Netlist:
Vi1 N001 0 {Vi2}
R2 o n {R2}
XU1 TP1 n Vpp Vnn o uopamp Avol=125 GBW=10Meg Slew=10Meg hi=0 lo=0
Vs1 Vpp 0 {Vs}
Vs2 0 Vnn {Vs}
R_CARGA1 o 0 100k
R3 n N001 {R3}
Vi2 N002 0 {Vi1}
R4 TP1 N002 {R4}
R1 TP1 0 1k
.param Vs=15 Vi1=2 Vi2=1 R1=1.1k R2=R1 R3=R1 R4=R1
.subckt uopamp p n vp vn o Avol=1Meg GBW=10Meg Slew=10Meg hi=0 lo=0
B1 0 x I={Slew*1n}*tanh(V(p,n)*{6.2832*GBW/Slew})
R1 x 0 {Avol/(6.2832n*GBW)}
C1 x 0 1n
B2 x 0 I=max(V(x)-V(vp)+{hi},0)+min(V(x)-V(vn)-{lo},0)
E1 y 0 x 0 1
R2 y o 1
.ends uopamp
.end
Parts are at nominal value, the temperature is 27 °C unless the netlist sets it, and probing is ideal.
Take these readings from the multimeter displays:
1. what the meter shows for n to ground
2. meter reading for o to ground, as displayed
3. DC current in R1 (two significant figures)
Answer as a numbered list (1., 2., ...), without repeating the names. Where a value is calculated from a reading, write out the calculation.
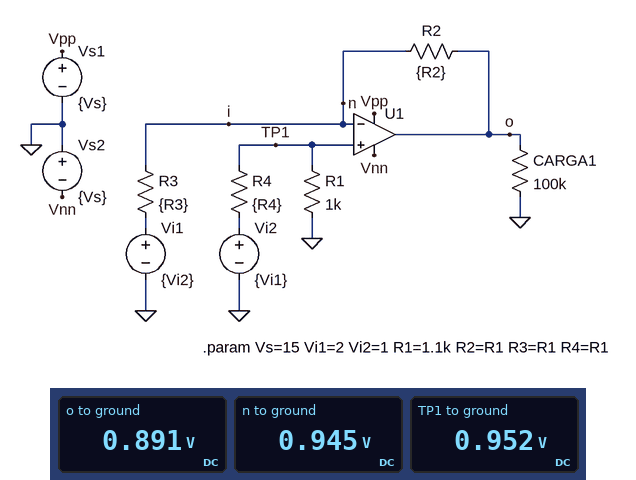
1. 0.945 V
2. 0.891 V
3. (952 mV) / 1 kΩ = 950 µA
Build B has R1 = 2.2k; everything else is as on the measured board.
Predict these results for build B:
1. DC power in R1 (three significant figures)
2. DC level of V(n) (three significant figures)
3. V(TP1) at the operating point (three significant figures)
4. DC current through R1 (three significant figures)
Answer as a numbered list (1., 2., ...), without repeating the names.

1. 808 µW
2. 1.32 V
3. 1.33 V
4. 606 µA
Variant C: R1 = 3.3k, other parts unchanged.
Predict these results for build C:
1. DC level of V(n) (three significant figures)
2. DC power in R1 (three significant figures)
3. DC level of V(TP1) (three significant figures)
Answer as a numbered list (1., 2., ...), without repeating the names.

1. 1.48 V
2. 682 µW
3. 1.50 V
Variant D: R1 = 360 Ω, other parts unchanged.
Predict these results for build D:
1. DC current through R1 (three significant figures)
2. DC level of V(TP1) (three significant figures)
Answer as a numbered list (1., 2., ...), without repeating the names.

1. 1.37 mA
2. 493 mV
